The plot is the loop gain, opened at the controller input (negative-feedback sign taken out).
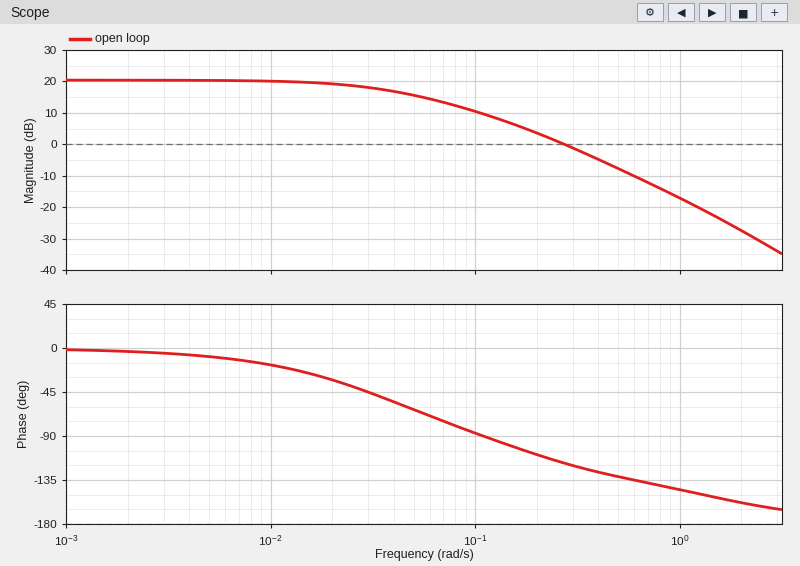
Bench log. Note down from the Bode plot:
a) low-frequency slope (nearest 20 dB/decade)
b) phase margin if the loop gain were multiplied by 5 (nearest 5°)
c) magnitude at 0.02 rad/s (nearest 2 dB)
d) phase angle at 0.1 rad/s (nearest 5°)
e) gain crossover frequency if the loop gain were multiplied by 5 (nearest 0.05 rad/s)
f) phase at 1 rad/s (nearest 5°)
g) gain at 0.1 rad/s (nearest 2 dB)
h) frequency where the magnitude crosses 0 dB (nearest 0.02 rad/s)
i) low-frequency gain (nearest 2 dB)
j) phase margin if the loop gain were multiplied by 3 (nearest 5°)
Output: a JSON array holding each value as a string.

["0 dB/decade", "40°", "20 dB", "-85°", "0.80 rad/s", "-145°", "10 dB", "0.28 rad/s", "20 dB", "45°"]
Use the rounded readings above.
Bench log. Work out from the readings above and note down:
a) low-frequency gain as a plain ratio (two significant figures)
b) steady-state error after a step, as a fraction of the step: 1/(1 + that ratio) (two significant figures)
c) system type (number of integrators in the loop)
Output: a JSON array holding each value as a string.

["10", "0.091", "0"]
